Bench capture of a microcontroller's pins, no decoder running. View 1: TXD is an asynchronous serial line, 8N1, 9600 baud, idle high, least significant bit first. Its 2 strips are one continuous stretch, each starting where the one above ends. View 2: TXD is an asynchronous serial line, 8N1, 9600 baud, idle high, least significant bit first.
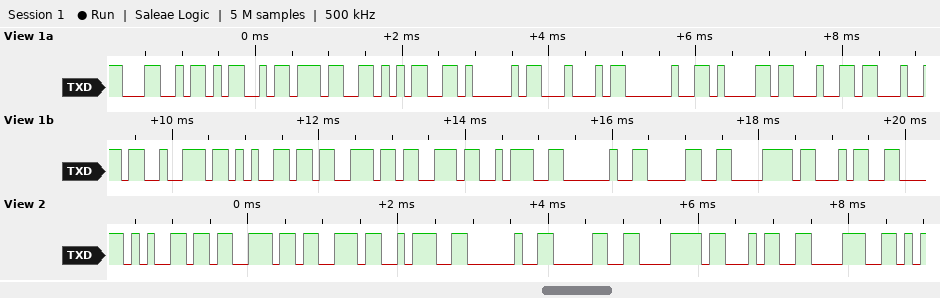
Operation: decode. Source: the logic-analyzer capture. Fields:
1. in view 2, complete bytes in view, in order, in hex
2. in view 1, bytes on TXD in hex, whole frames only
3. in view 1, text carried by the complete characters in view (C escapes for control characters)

65 73 73 3A 20 30 78 34 38
4C 4D 37 35 41 44 20 61 64 64 72 65 73 73 3A 20 30 78 34
"LM75AD address: 0x4"
